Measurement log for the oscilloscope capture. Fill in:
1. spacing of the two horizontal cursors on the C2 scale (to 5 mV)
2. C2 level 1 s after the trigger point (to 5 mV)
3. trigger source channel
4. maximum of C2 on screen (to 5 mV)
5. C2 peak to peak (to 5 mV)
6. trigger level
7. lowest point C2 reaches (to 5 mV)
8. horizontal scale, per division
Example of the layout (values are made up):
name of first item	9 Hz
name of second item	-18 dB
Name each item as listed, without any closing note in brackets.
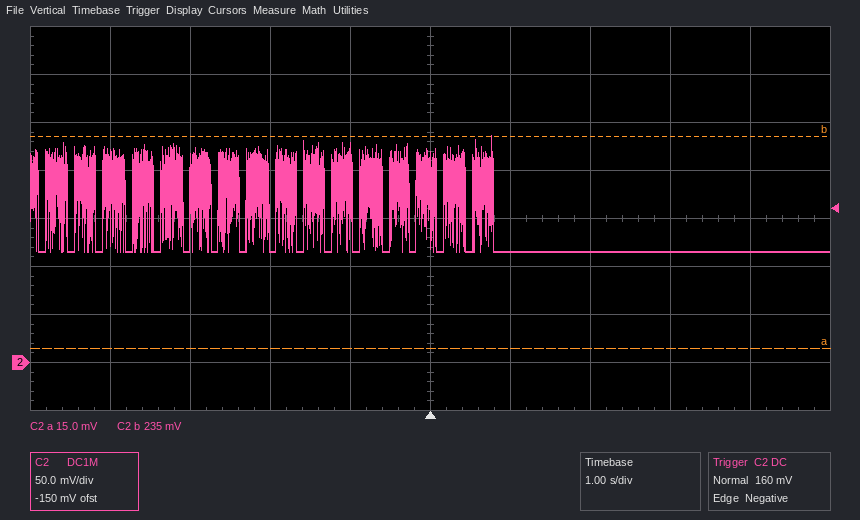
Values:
spacing of the two horizontal cursors on the C2 scale	220 mV
C2 level 1 s after the trigger point	115 mV
trigger source channel	C2
maximum of C2 on screen	235 mV
C2 peak to peak	120 mV
trigger level	160 mV
lowest point C2 reaches	115 mV
horizontal scale, per division	1 s
